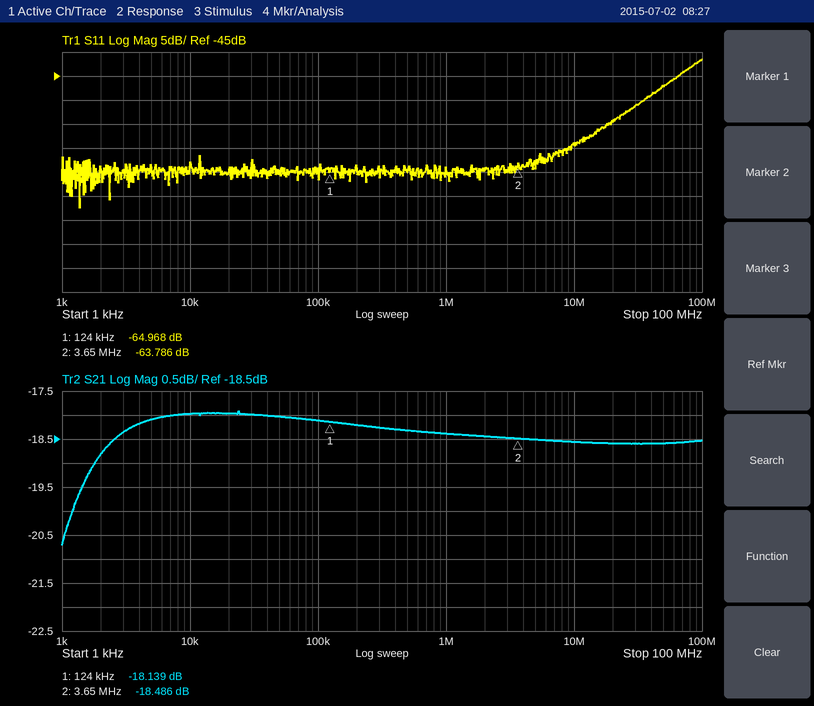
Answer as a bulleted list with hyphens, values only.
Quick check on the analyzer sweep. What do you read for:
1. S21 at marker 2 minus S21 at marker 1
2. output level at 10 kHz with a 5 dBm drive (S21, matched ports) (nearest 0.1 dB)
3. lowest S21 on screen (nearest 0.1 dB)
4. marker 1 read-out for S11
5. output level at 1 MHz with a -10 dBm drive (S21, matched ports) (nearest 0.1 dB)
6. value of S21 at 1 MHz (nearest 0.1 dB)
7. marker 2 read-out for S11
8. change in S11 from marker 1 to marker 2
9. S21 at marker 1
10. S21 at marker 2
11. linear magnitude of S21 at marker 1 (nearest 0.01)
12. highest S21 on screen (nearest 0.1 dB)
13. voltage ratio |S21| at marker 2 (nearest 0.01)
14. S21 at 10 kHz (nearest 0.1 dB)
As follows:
- -0.347 dB
- -13.0 dBm
- -20.7 dB
- -64.968 dB
- -28.4 dBm
- -18.4 dB
- -63.786 dB
- 1.182 dB
- -18.139 dB
- -18.486 dB
- 0.12
- -17.9 dB
- 0.12
- -18.0 dB
